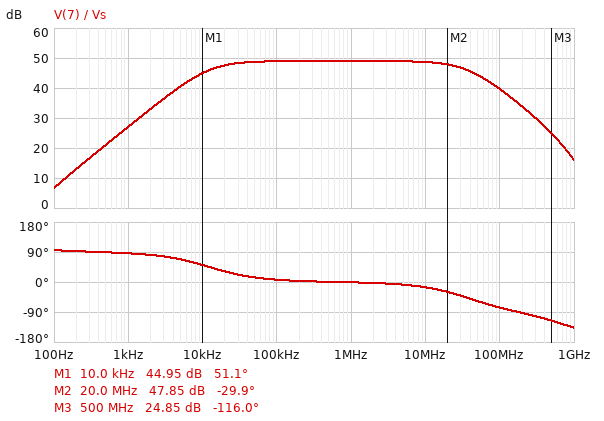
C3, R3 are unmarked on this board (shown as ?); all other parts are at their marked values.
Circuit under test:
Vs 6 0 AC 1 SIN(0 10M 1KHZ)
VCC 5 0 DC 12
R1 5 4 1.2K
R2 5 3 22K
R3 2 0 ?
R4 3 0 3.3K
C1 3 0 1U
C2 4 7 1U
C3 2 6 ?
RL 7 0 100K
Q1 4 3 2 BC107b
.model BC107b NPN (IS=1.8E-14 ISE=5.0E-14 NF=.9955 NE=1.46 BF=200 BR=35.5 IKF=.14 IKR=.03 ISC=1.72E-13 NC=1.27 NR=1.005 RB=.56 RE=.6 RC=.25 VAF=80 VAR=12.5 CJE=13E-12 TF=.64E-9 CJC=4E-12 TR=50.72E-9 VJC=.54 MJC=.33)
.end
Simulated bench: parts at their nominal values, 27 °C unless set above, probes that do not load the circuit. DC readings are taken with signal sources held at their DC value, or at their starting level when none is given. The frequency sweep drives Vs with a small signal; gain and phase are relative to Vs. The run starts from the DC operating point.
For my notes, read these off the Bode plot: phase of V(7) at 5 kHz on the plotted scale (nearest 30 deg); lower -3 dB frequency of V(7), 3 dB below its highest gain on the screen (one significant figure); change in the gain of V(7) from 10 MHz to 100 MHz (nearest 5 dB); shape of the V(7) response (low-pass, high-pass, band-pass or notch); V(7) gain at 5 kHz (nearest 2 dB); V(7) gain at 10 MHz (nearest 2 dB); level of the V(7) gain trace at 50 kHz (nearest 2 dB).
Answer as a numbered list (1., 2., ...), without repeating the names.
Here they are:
1. 60 deg
2. 10 kHz
3. -10 dB
4. band-pass
5. 40 dB
6. 48 dB
7. 48 dB
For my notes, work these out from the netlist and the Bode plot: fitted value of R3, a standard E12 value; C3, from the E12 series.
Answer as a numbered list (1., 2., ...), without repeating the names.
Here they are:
1. 82 Ω
2. 3.3 µF
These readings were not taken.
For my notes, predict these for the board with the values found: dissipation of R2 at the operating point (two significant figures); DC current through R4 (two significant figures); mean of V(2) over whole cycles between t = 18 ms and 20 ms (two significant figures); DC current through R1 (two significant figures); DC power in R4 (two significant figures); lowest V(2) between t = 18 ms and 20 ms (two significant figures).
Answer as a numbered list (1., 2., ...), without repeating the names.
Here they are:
1. 5.1 mW
2. 430 µA
3. 710 mV
4. 8.6 mA
5. 600 µW
6. 710 mV
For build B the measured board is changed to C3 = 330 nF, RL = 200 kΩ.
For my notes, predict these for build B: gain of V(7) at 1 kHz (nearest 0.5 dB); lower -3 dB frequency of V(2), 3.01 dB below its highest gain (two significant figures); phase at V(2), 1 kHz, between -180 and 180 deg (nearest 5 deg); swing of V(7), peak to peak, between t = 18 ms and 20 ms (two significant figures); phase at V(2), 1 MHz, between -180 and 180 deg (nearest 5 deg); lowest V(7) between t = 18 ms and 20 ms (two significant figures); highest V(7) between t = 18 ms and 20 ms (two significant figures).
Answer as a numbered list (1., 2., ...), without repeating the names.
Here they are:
1. 7.5 dB
2. 120 kHz
3. 75 deg
4. 47 mV
5. 5 deg
6. -23 mV
7. 23 mV
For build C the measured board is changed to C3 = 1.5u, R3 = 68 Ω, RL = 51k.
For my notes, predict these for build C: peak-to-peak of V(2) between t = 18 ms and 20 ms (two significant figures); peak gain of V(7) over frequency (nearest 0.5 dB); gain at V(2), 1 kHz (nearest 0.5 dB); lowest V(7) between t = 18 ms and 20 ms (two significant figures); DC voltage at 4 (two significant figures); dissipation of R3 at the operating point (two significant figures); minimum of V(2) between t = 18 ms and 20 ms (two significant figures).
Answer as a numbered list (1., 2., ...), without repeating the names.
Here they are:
1. 5.8 mV
2. 32.5 dB
3. -10.5 dB
4. -26 mV
5. 760 mV
6. 6.1 mW
7. 640 mV
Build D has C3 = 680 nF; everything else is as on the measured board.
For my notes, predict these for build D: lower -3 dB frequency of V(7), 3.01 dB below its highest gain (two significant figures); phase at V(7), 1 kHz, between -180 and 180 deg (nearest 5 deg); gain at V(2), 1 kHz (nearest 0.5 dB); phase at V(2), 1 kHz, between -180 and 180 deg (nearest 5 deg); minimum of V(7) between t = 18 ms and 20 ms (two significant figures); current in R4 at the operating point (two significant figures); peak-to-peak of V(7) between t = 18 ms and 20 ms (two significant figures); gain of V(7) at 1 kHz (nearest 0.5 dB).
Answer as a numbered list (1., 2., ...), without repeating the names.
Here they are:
1. 59 kHz
2. 90 deg
3. -35.0 dB
4. 75 deg
5. -48 mV
6. 430 µA
7. 95 mV
8. 13.5 dB
